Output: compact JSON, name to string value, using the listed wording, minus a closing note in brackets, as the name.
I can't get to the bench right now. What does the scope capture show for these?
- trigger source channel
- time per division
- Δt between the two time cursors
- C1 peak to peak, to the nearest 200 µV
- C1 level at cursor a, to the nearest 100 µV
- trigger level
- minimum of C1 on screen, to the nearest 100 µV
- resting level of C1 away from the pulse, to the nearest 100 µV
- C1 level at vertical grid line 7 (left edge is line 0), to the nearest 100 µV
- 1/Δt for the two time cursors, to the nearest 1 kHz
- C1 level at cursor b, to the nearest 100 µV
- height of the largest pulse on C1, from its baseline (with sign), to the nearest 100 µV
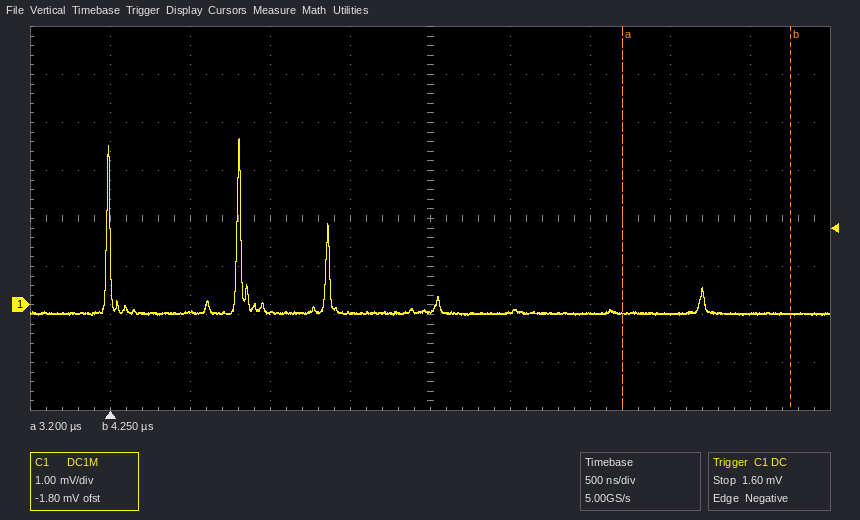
{"trigger source channel": "C1", "time per division": "500 ns", "Δt between the two time cursors": "1.05 µs", "C1 peak to peak, to the nearest 200 µV": "3.6 mV", "C1 level at cursor a, to the nearest 100 µV": "-200 µV", "trigger level": "1.60 mV", "minimum of C1 on screen, to the nearest 100 µV": "-200 µV", "resting level of C1 away from the pulse, to the nearest 100 µV": "-200 µV", "C1 level at vertical grid line 7 (left edge is line 0), to the nearest 100 µV": "-200 µV", "1/Δt for the two time cursors, to the nearest 1 kHz": "952 kHz", "C1 level at cursor b, to the nearest 100 µV": "-200 µV", "height of the largest pulse on C1, from its baseline (with sign), to the nearest 100 µV": "+3.6 mV"}
